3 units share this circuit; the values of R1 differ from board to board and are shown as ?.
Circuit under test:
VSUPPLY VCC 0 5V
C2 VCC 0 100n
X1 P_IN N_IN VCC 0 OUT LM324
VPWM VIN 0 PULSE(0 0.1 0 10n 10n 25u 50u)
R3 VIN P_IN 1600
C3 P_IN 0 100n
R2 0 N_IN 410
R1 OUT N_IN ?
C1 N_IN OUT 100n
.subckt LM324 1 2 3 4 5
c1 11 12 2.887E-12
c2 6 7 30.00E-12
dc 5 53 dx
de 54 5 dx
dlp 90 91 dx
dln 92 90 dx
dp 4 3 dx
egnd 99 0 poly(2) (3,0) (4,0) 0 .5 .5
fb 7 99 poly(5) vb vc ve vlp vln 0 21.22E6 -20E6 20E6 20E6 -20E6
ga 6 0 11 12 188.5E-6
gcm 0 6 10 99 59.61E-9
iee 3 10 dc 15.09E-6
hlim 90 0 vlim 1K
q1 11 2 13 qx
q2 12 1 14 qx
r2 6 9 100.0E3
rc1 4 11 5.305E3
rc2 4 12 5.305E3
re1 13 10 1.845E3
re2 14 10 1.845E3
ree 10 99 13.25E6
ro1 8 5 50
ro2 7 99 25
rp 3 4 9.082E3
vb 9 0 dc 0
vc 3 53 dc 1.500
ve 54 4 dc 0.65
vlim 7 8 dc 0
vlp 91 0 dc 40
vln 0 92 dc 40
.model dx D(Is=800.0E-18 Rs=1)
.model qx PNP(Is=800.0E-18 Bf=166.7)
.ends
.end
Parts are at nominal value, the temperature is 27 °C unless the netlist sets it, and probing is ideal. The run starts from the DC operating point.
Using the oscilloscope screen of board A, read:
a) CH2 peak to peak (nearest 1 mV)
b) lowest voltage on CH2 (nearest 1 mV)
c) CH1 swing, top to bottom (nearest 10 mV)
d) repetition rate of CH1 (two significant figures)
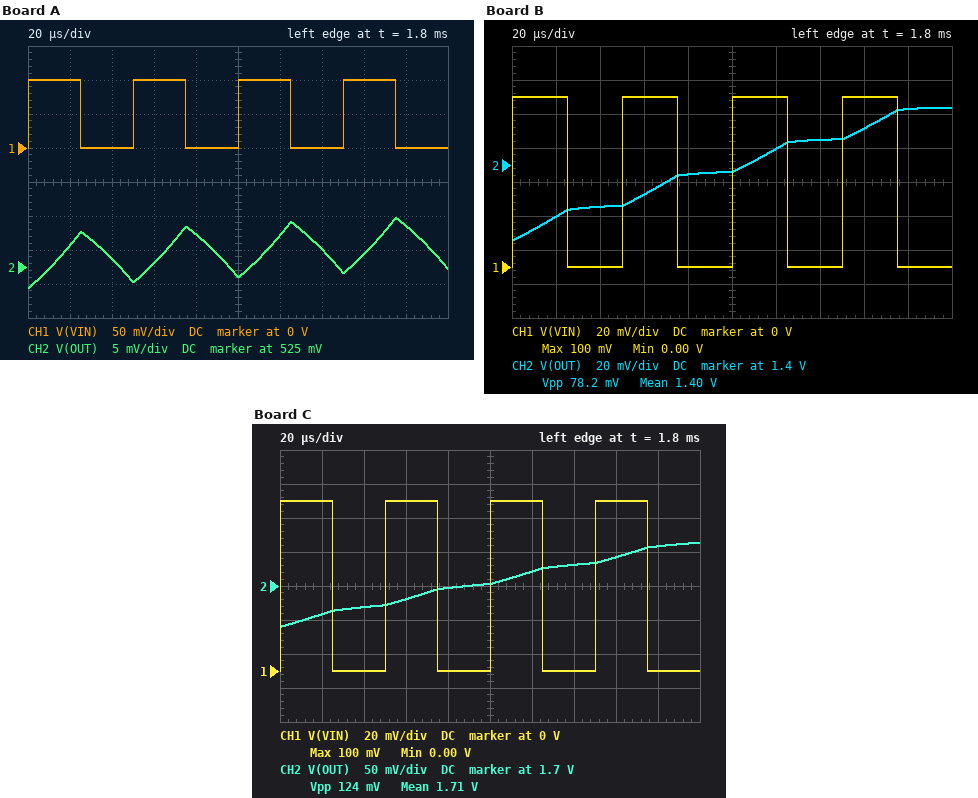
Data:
10 mV
522 mV
100 mV
20 kHz
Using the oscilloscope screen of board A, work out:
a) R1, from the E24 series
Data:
3.9 kΩ
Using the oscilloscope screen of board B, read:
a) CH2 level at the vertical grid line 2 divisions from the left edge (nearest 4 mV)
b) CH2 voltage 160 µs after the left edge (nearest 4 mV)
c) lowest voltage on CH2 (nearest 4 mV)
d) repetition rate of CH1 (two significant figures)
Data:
1.376 V
1.420 V
1.356 V
20 kHz
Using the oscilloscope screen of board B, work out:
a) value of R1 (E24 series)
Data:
16 kΩ
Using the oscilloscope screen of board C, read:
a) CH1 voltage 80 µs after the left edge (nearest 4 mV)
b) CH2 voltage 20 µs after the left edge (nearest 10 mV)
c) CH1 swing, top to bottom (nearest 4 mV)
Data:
0 V
1.66 V
100 mV
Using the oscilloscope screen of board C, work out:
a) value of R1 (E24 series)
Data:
27 kΩ
